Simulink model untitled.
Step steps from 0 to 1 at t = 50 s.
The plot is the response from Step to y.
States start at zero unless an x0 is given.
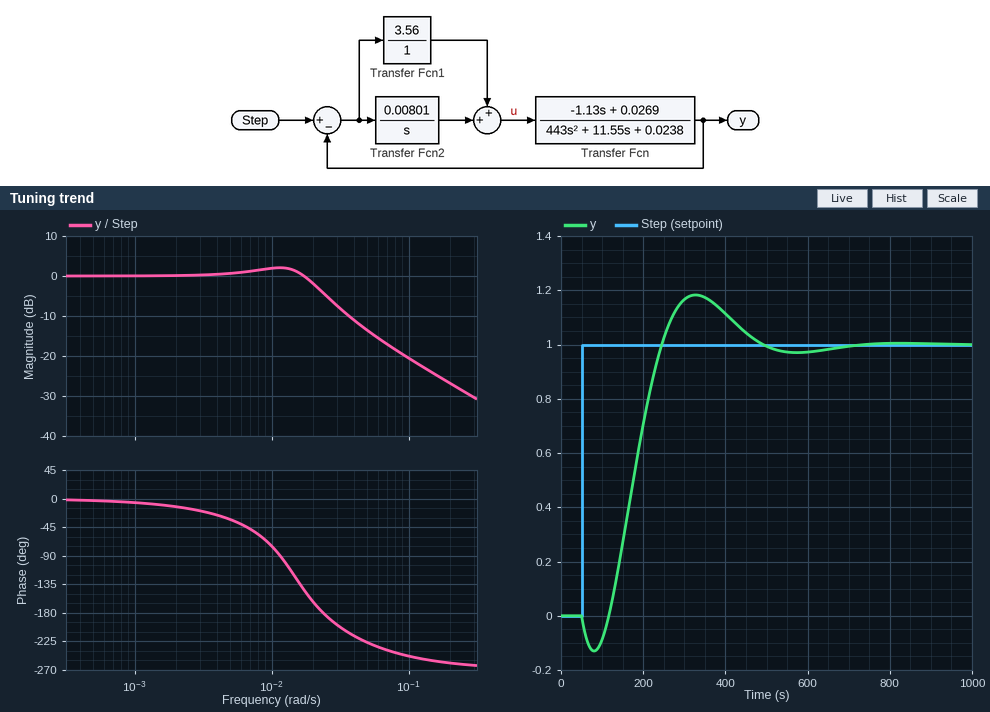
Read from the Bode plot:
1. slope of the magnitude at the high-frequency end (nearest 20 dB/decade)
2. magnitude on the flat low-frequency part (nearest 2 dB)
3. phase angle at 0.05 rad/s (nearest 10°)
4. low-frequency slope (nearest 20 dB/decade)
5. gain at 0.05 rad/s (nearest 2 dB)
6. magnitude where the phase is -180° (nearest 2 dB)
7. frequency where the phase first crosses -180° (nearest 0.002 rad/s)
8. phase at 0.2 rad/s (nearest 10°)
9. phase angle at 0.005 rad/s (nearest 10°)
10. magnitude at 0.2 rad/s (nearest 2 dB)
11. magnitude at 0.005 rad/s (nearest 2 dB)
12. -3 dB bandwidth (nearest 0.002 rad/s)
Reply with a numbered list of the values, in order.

1. -20 dB/decade
2. 0 dB
3. -230°
4. 0 dB/decade
5. -14 dB
6. -4 dB
7. 0.024 rad/s
8. -260°
9. -30°
10. -26 dB
11. 0 dB
12. 0.022 rad/s
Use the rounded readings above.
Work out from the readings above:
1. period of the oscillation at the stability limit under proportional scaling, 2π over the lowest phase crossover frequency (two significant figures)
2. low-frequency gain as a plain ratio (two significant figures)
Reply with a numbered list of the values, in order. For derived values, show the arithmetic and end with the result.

1. 2π / 0.024 = 260 s
2. 10^(0 / 20) = 1.0
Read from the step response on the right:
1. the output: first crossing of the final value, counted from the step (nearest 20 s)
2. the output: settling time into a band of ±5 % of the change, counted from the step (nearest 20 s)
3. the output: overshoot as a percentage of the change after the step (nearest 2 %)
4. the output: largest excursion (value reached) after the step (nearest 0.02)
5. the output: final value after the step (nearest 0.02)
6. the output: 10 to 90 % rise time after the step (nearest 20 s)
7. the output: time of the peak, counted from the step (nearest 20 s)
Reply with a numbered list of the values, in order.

1. 200 s
2. 400 s
3. 18 %
4. 1.18
5. 1.00
6. 100 s
7. 280 s
